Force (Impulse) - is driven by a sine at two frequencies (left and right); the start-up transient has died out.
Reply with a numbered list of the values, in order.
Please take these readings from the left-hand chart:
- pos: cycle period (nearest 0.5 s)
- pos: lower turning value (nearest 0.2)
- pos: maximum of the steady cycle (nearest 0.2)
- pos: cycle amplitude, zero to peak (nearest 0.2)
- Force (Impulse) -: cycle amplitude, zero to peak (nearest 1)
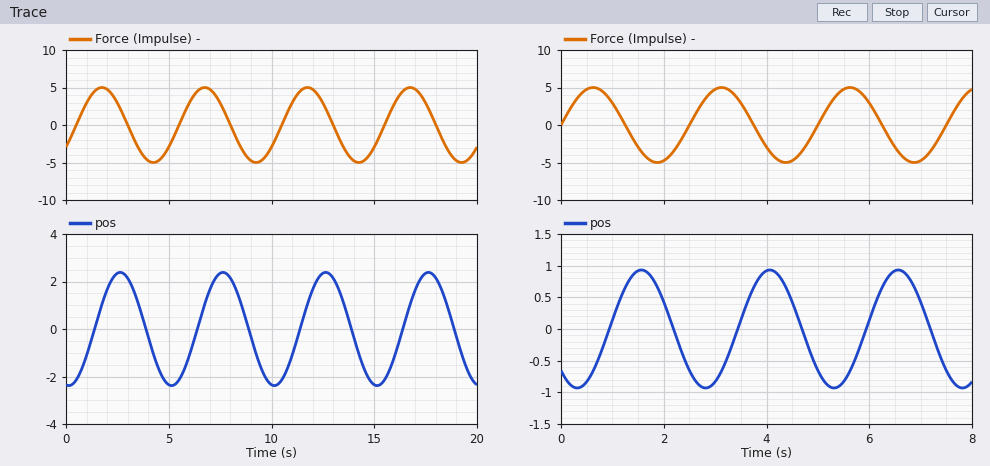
1. 5.0 s
2. -2.4
3. 2.4
4. 2.4
5. 5
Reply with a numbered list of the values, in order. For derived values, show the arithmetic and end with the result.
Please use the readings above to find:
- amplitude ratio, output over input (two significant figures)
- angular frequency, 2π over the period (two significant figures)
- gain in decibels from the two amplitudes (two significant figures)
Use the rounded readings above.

1. 2.4 / 5 = 0.48
2. 2π / 5 = 1.3 rad/s
3. 20 log10(2.4 / 5) = -6.4 dB
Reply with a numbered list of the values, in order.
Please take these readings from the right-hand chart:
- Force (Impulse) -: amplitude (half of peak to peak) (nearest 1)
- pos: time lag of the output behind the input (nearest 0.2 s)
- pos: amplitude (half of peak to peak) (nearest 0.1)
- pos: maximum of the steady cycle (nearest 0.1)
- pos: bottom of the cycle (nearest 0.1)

1. 5
2. 1.0 s
3. 0.9
4. 0.9
5. -0.9
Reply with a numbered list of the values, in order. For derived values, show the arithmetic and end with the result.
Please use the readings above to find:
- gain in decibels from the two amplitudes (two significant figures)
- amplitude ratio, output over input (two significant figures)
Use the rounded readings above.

1. 20 log10(0.9 / 5) = -15 dB
2. 0.9 / 5 = 0.18
